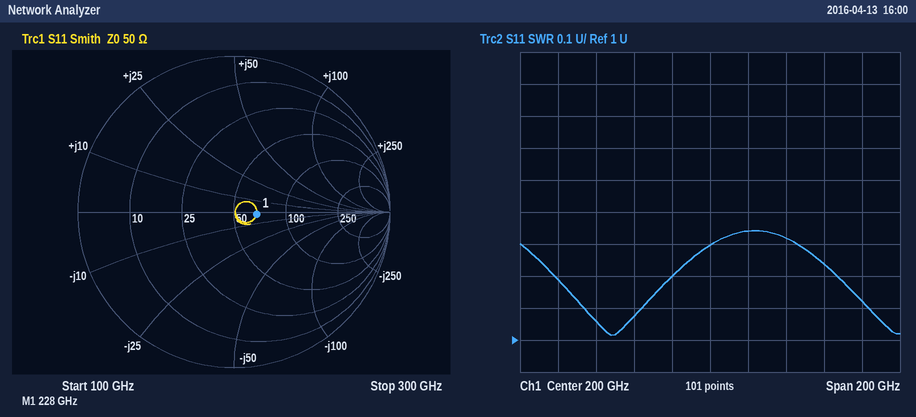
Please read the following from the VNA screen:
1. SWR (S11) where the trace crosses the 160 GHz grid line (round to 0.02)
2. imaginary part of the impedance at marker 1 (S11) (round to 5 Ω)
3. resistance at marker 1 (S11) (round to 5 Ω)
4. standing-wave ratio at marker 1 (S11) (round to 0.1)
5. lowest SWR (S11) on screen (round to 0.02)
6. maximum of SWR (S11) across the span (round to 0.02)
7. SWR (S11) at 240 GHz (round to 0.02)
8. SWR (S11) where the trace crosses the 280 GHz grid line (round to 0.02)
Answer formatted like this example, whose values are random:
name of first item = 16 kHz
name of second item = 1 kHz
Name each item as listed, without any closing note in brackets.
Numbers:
SWR (S11) where the trace crosses the 160 GHz grid line = 1.08
imaginary part of the impedance at marker 1 (S11) = 0 Ω
resistance at marker 1 (S11) = 65 Ω
standing-wave ratio at marker 1 (S11) = 1.3
lowest SWR (S11) on screen = 1.02
maximum of SWR (S11) across the span = 1.34
SWR (S11) at 240 GHz = 1.32
SWR (S11) where the trace crosses the 280 GHz grid line = 1.12
